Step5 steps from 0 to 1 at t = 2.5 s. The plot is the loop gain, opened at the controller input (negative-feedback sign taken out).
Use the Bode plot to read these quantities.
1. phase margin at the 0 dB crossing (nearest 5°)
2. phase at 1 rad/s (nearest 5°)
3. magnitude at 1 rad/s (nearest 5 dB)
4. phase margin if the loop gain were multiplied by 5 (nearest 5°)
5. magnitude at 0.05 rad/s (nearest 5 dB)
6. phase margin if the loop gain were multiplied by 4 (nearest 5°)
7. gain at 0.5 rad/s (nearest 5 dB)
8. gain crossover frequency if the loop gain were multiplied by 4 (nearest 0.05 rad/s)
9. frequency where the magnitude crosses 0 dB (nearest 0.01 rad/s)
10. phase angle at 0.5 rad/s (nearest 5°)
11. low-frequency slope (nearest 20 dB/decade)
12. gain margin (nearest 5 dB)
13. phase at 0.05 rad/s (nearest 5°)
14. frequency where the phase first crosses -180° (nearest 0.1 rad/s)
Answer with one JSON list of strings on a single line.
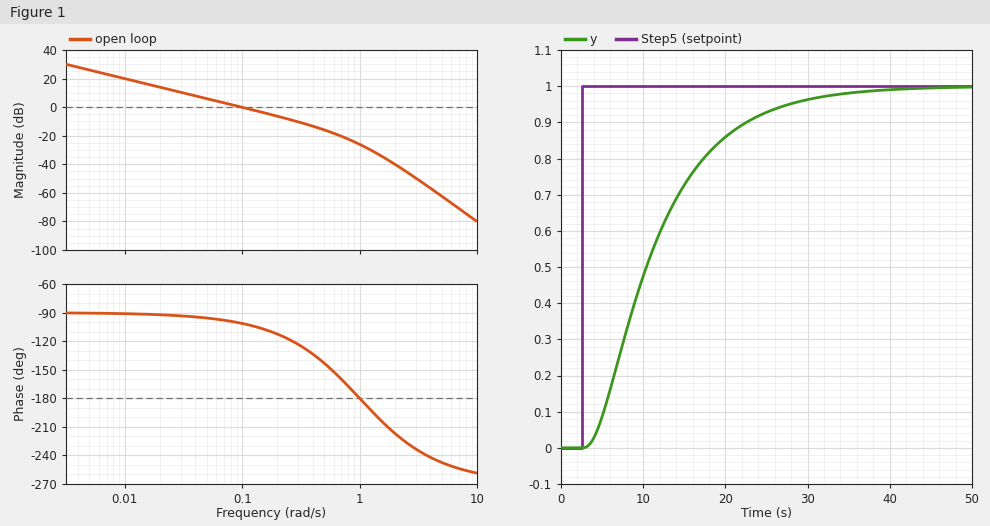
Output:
["80°", "-180°", "-25 dB", "45°", "5 dB", "50°", "-15 dB", "0.35 rad/s", "0.10 rad/s", "-145°", "-20 dB/decade", "25 dB", "-95°", "1.0 rad/s"]
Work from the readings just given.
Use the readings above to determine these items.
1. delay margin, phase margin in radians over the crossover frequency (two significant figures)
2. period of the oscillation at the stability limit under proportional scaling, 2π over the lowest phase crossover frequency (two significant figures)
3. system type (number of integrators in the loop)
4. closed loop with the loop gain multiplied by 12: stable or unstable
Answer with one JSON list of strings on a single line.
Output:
["14 s", "6.3 s", "1", "stable"]
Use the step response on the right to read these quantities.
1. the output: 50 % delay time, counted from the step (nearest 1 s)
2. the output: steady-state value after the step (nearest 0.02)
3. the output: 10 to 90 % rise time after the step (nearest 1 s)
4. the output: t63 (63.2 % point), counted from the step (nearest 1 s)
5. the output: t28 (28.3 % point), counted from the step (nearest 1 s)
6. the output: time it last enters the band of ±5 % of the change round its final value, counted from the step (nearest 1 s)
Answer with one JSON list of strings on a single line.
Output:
["8 s", "1.00", "17 s", "10 s", "5 s", "25 s"]
